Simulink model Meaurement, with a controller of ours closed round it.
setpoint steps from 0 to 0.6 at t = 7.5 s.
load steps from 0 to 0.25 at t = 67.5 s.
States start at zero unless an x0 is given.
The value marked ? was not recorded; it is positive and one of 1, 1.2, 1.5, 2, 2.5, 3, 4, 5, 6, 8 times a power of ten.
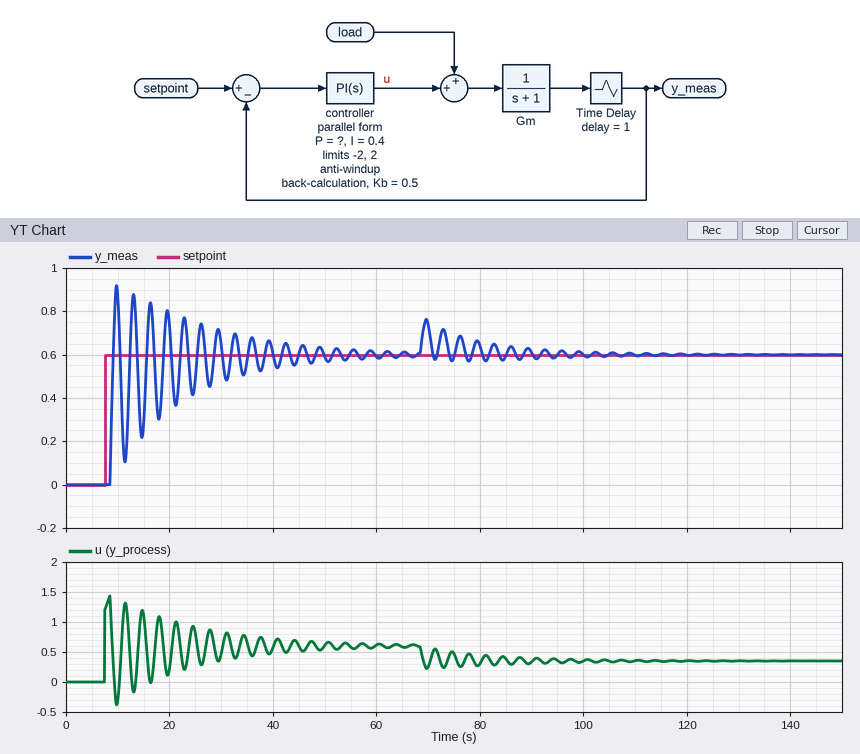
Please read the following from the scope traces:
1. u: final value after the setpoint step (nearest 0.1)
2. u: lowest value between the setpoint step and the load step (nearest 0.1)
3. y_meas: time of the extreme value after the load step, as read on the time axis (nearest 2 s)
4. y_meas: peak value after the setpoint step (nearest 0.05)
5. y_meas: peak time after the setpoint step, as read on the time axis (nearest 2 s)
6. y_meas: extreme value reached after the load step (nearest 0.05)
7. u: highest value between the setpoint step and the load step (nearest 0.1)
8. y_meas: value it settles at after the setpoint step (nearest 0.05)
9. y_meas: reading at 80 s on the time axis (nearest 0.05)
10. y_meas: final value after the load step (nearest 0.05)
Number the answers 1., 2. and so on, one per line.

1. 0.6
2. -0.4
3. 70 s
4. 0.90
5. 10 s
6. 0.75
7. 1.4
8. 0.60
9. 0.65
10. 0.60
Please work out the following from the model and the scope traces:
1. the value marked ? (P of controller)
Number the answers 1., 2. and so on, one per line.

1. 2
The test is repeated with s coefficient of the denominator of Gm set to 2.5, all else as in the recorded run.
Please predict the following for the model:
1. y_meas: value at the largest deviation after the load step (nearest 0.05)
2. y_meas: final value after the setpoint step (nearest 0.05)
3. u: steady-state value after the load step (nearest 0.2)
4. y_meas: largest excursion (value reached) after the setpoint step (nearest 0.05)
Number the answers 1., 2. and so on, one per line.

1. 0.70
2. 0.60
3. 0.4
4. 0.65
